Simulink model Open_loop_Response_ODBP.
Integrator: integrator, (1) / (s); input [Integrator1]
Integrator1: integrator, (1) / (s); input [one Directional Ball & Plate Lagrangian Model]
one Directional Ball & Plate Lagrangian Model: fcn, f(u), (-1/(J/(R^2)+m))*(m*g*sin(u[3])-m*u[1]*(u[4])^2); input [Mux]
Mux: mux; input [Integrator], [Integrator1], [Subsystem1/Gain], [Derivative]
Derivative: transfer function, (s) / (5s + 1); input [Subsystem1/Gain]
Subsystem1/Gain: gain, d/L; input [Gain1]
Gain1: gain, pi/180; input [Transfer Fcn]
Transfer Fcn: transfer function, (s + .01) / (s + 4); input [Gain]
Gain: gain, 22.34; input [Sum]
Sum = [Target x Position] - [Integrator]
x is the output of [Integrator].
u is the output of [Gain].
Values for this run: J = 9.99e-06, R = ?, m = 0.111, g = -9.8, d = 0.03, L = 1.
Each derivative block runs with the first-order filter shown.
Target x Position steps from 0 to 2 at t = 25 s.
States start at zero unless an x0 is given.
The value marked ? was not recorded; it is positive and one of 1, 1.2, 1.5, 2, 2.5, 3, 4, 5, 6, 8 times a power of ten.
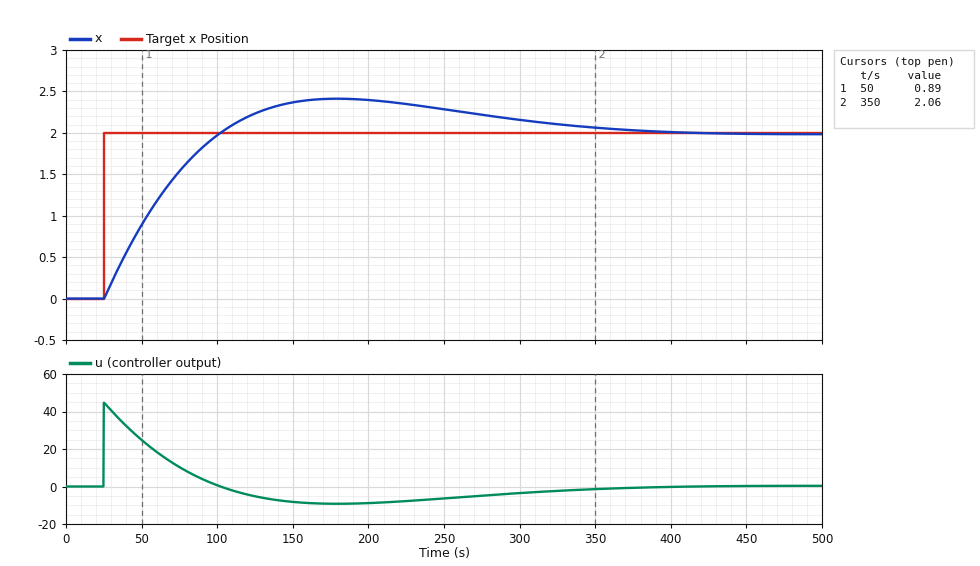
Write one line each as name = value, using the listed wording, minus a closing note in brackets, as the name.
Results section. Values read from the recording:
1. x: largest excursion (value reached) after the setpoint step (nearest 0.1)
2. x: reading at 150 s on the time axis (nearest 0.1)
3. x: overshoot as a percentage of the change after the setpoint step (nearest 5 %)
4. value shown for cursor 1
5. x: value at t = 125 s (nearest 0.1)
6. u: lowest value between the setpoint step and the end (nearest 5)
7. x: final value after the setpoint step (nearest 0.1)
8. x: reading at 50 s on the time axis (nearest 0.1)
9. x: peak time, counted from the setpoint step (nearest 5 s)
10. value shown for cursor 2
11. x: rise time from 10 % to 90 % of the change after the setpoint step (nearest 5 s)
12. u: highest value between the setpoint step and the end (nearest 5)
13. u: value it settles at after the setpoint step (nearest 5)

x: largest excursion (value reached) after the setpoint step = 2.4
x: reading at 150 s on the time axis = 2.4
x: overshoot as a percentage of the change after the setpoint step = 20 %
value shown for cursor 1 = 0.89
x: value at t = 125 s = 2.2
u: lowest value between the setpoint step and the end = -10
x: final value after the setpoint step = 2.0
x: reading at 50 s on the time axis = 0.9
x: peak time, counted from the setpoint step = 155 s
value shown for cursor 2 = 2.06
x: rise time from 10 % to 90 % of the change after the setpoint step = 60 s
u: highest value between the setpoint step and the end = 45
u: value it settles at after the setpoint step = 0
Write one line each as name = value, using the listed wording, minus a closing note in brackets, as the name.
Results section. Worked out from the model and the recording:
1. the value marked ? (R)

the value marked ? = 0.015
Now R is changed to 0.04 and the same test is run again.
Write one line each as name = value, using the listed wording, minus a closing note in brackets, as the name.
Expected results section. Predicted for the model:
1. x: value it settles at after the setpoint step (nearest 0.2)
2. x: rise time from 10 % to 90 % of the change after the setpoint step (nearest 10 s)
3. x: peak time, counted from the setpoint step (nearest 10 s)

x: value it settles at after the setpoint step = 2.0
x: rise time from 10 % to 90 % of the change after the setpoint step = 50 s
x: peak time, counted from the setpoint step = 130 s
